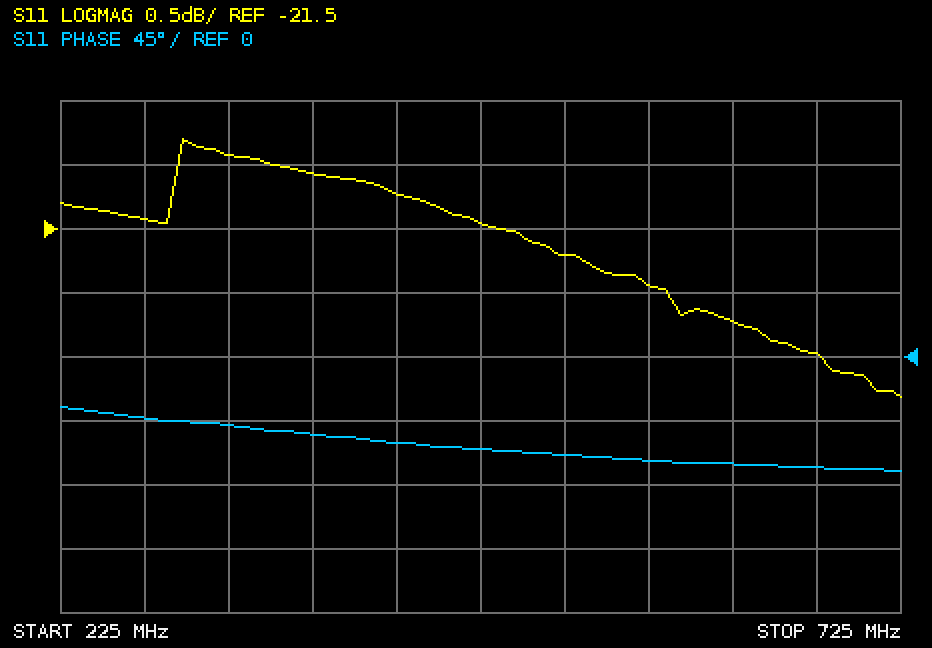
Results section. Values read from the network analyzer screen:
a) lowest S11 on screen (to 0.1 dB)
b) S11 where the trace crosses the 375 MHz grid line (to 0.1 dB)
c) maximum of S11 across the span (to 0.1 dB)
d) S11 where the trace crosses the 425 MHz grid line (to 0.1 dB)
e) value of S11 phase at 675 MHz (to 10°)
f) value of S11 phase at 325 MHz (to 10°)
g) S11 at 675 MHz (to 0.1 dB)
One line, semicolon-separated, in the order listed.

-22.8 dB; -21.1 dB; -20.8 dB; -21.2 dB; -80°; -50°; -22.5 dB
